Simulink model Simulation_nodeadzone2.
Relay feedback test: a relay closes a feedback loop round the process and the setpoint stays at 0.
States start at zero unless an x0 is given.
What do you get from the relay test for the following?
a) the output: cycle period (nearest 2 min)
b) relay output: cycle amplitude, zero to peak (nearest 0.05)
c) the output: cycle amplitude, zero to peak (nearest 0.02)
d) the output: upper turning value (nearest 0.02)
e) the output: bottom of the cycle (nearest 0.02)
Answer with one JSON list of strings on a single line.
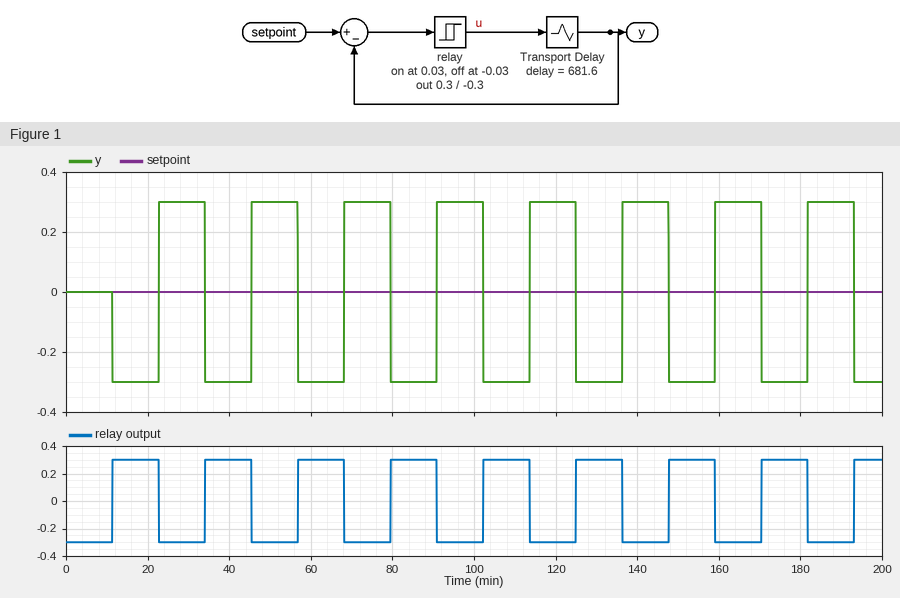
["22 min", "0.30", "0.30", "0.30", "-0.30"]
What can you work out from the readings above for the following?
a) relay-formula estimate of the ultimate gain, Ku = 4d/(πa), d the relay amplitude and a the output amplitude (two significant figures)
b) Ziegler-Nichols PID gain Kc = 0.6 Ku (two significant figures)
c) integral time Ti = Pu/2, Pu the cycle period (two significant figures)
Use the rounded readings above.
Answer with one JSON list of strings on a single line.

["1.3", "0.78", "11 min"]
